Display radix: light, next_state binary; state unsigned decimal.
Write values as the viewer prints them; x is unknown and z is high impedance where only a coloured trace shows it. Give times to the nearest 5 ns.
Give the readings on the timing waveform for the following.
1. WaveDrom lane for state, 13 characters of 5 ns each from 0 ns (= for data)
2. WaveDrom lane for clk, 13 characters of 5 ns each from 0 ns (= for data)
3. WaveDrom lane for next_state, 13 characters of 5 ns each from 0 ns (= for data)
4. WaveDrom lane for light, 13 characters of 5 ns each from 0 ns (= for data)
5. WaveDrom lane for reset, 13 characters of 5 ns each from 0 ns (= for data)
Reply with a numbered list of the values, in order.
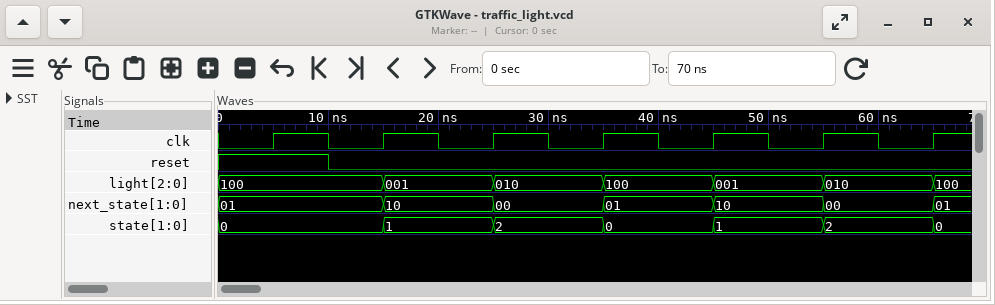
1. {name: 'state', wave: '=..=.=.=.=.=.', data: '0 1 2 0 1 2'}
2. {name: 'clk', wave: '0101010101010'}
3. {name: 'next_state', wave: '=..=.=.=.=.=.', data: '01 10 00 01 10 00'}
4. {name: 'light', wave: '=..=.=.=.=.=.', data: '100 001 010 100 001 010'}
5. {name: 'reset', wave: '1.0..........'}
